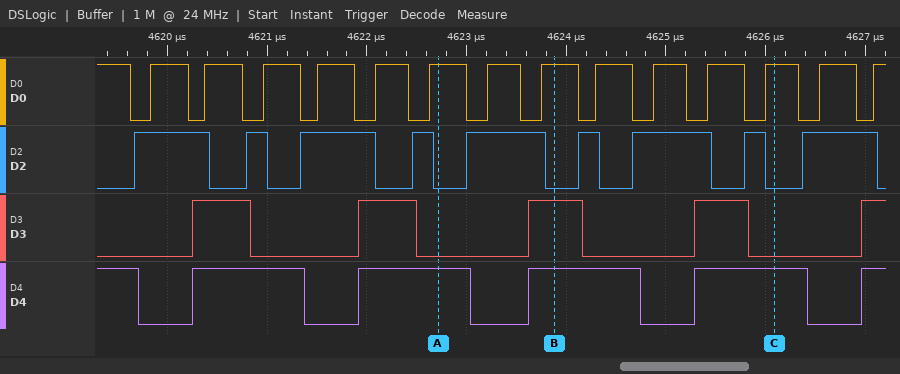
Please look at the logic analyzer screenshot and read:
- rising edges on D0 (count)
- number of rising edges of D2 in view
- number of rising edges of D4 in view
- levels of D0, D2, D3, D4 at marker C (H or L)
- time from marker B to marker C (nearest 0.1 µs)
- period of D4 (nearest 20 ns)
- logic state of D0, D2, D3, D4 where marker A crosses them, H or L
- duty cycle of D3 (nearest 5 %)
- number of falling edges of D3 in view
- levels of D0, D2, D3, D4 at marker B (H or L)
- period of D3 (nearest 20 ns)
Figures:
14
9
5
D0=H, D2=L, D3=L, D4=H
2.2 µs
1680 ns
D0=H, D2=L, D3=L, D4=H
35 %
4
D0=H, D2=L, D3=H, D4=H
1680 ns
